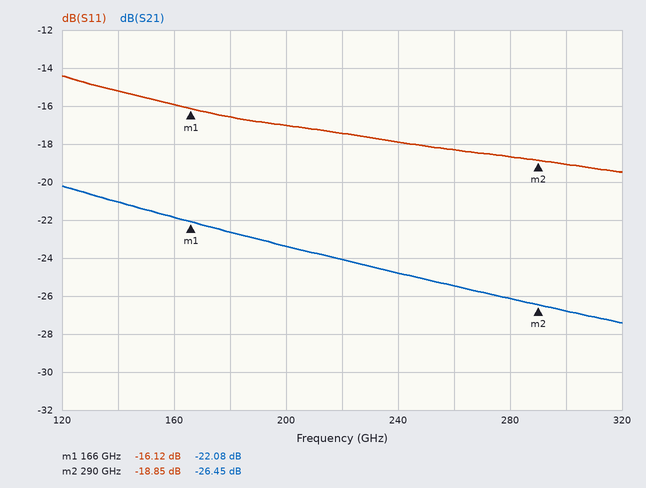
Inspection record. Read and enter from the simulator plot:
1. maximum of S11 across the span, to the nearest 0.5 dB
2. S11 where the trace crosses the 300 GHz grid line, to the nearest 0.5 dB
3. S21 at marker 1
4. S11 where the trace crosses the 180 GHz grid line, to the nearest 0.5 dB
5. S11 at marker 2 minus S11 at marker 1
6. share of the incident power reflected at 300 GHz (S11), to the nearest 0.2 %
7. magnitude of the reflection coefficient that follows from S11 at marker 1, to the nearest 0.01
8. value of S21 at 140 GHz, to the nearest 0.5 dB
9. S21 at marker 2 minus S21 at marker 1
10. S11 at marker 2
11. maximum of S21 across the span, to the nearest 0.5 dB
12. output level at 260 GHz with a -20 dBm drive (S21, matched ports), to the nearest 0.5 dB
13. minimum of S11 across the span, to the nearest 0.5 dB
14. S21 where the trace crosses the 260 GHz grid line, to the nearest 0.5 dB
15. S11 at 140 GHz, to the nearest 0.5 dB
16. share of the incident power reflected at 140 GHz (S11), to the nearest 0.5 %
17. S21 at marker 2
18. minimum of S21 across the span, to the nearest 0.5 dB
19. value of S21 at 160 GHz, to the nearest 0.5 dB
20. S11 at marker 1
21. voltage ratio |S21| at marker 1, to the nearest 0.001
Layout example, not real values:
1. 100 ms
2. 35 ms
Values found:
1. -14.5 dB
2. -19.0 dB
3. -22.08 dB
4. -16.5 dB
5. -2.73 dB
6. 1.2 %
7. 0.16
8. -21.0 dB
9. -4.37 dB
10. -18.85 dB
11. -20.0 dB
12. -45.5 dBm
13. -19.5 dB
14. -25.5 dB
15. -15.0 dB
16. 3.0 %
17. -26.45 dB
18. -27.5 dB
19. -22.0 dB
20. -16.12 dB
21. 0.079
